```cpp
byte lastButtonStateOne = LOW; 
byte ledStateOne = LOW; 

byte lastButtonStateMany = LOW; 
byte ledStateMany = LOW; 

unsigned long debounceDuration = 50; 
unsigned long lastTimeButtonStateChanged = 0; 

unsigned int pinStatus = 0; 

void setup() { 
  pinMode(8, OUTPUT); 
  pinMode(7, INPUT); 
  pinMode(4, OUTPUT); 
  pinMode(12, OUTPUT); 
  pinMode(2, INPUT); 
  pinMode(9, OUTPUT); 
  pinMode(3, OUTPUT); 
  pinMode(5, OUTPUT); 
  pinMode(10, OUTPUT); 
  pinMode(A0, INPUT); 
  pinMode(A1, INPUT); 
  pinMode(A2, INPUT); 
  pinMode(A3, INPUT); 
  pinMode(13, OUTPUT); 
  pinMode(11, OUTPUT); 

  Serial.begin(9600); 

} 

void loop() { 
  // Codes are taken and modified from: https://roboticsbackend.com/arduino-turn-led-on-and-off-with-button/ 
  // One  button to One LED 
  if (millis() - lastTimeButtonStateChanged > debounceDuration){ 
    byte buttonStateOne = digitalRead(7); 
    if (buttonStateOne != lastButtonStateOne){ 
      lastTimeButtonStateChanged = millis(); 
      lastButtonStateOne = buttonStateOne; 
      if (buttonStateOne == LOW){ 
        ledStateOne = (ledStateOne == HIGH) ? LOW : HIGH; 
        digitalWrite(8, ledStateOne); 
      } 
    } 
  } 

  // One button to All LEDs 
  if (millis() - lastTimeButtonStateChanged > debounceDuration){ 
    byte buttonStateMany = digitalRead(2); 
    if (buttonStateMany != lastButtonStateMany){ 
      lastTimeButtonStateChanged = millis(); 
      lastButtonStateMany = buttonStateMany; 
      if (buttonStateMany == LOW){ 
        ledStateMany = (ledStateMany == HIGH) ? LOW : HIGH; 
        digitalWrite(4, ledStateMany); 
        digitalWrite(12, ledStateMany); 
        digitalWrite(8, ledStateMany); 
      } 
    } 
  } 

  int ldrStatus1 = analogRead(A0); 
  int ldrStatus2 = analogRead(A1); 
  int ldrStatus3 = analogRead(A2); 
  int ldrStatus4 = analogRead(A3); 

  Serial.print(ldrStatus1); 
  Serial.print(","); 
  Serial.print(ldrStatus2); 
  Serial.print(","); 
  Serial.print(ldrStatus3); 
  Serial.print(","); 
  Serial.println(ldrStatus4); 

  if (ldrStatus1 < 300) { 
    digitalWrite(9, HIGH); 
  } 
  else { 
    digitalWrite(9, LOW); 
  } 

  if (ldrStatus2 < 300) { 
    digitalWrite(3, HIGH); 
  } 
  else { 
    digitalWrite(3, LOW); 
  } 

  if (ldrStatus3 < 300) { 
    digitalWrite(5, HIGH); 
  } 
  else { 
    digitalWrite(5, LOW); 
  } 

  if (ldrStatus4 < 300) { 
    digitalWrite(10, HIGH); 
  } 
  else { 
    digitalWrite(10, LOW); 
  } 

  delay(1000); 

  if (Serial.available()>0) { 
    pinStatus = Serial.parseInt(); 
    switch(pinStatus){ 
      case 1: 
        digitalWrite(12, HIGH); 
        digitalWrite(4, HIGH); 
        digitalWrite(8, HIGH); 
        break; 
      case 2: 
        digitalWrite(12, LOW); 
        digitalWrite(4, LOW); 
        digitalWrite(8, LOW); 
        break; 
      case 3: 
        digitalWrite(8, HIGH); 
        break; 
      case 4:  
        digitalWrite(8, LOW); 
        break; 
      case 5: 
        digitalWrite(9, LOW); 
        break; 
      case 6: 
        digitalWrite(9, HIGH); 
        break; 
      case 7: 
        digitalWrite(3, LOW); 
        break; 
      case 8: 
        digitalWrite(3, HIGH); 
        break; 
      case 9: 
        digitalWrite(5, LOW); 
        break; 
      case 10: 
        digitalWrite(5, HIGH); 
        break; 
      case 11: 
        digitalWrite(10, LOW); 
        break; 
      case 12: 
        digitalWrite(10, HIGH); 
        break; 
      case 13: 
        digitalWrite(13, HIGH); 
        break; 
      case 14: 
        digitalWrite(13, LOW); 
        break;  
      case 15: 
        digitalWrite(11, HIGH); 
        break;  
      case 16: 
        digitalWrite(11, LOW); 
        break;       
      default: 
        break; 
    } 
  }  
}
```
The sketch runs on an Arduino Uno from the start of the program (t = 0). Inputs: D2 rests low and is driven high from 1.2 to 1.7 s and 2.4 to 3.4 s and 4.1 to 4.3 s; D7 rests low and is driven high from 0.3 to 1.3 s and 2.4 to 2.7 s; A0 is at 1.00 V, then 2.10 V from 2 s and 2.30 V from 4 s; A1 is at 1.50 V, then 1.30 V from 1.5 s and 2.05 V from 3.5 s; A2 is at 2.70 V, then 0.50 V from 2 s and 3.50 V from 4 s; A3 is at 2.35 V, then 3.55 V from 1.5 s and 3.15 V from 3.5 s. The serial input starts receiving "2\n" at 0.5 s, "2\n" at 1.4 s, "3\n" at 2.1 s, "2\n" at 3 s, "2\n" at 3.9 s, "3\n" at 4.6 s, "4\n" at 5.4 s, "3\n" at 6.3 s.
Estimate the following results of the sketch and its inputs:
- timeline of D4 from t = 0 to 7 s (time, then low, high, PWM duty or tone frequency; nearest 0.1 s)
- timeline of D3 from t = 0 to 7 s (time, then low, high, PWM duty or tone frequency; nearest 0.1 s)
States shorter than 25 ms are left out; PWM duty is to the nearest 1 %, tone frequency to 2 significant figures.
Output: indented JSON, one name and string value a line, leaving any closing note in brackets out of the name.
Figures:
{
  "timeline of D4 from t = 0 to 7 s": "0 s low; 4 s high; 5 s low",
  "timeline of D3 from t = 0 to 7 s": "0 s low; 2 s high; 4 s low"
}
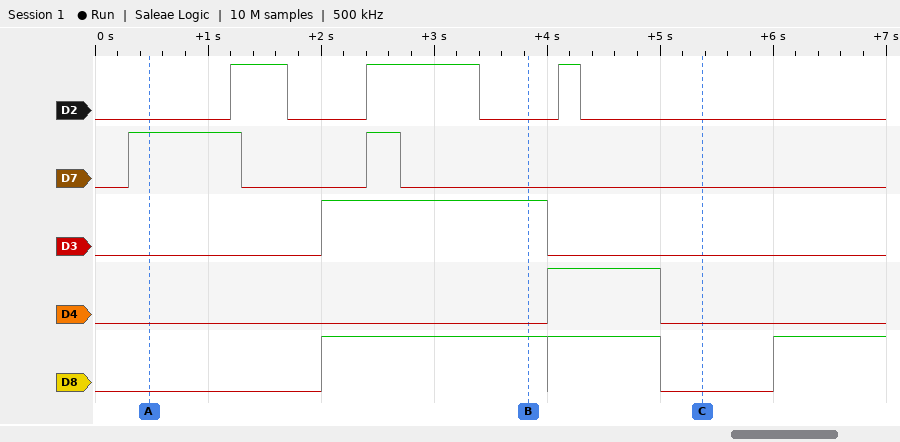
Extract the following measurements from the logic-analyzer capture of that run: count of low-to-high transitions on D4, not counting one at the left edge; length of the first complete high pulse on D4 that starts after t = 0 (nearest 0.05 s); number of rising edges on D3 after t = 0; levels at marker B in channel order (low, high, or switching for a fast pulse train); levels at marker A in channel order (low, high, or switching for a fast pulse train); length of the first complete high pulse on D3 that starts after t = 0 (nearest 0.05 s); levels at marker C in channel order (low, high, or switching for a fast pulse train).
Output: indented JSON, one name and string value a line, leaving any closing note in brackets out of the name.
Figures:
{
  "count of low-to-high transitions on D4, not counting one at the left edge": "1",
  "length of the first complete high pulse on D4 that starts after t = 0": "1.00 s",
  "number of rising edges on D3 after t = 0": "1",
  "levels at marker B in channel order": "D2 low, D7 low, D3 high, D4 low, D8 high",
  "levels at marker A in channel order": "D2 low, D7 high, D3 low, D4 low, D8 low",
  "length of the first complete high pulse on D3 that starts after t = 0": "2.00 s",
  "levels at marker C in channel order": "D2 low, D7 low, D3 low, D4 low, D8 low"
}
